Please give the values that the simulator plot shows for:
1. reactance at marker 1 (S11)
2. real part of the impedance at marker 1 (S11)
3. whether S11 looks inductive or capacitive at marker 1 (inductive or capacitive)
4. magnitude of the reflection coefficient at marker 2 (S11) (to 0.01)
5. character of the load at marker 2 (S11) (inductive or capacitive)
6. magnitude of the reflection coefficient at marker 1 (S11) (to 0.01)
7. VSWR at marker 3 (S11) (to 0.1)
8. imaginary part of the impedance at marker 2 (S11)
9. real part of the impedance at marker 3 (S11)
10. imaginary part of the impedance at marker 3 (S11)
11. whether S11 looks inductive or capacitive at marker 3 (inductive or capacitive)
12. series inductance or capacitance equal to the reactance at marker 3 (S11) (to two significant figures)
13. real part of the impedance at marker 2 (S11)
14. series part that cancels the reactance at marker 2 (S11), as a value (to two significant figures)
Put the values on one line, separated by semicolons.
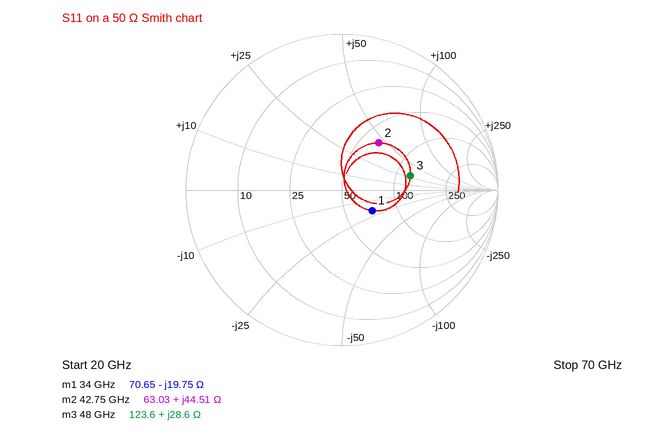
-19.75 Ω; 70.65 Ω; capacitive; 0.38; inductive; 0.23; 2.6; +44.51 Ω; 123.6 Ω; +28.6 Ω; inductive; 95 pH; 63.03 Ω; 84 fF
